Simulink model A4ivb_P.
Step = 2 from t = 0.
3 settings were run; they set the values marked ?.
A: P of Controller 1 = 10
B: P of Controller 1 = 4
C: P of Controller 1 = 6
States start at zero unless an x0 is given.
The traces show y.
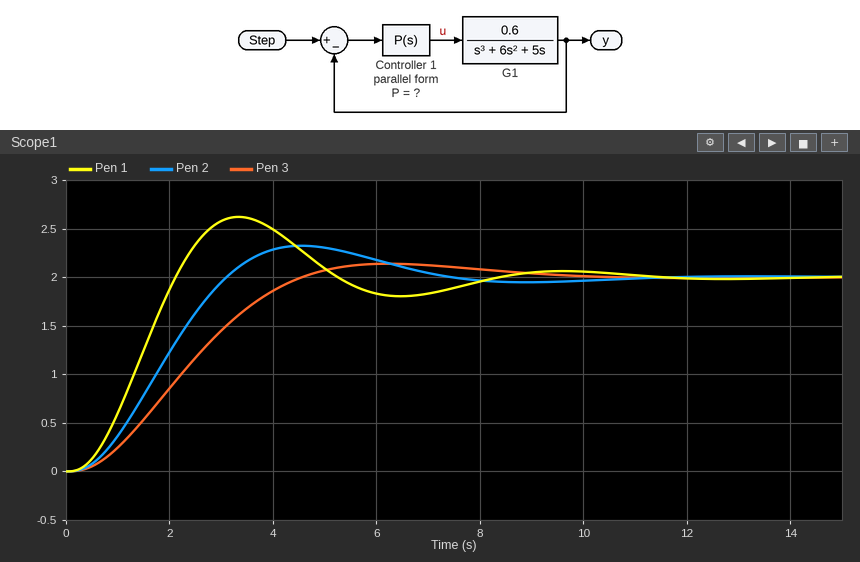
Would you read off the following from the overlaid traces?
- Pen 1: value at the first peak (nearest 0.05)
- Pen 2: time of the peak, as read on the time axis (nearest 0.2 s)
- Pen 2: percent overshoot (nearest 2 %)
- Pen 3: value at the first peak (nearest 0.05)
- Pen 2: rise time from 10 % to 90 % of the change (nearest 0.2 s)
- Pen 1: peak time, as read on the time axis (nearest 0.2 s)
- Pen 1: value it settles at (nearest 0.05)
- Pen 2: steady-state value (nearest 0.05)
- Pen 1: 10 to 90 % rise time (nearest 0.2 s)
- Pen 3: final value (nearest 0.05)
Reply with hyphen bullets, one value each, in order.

- 2.60
- 4.6 s
- 16 %
- 2.15
- 2.0 s
- 3.4 s
- 2.00
- 2.00
- 1.4 s
- 2.00
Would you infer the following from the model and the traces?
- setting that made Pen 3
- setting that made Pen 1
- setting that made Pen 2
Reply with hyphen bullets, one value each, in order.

- B
- A
- C
